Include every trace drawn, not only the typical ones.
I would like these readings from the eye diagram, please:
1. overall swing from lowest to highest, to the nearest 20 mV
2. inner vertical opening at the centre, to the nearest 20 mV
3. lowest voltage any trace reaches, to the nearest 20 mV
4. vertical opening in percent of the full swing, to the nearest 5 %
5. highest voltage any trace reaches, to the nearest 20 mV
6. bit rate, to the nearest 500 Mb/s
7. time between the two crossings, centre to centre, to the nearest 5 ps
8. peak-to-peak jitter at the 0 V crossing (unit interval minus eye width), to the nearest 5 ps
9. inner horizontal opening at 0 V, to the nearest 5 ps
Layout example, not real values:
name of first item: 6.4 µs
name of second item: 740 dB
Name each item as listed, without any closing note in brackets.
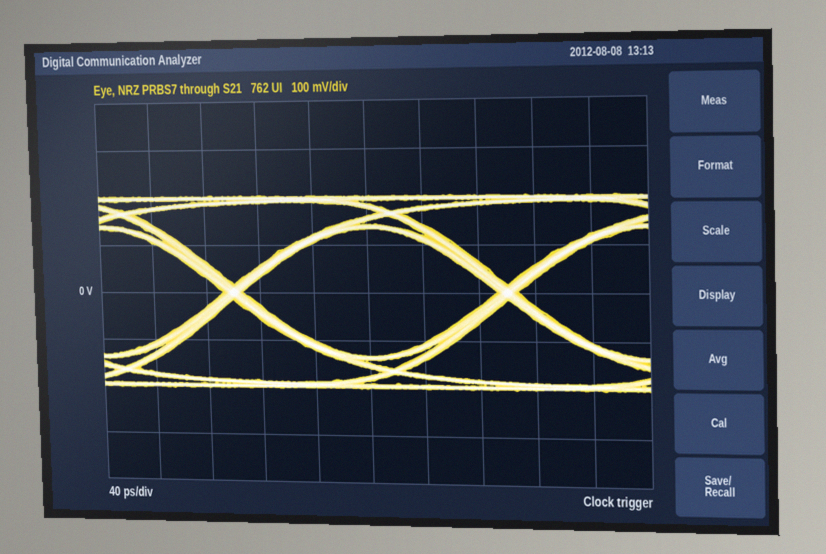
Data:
overall swing from lowest to highest, to the nearest 20 mV: 400 mV
inner vertical opening at the centre, to the nearest 20 mV: 260 mV
lowest voltage any trace reaches, to the nearest 20 mV: -200 mV
vertical opening in percent of the full swing, to the nearest 5 %: 65 %
highest voltage any trace reaches, to the nearest 20 mV: 200 mV
bit rate, to the nearest 500 Mb/s: 5.0 Gb/s
time between the two crossings, centre to centre, to the nearest 5 ps: 200 ps
peak-to-peak jitter at the 0 V crossing (unit interval minus eye width), to the nearest 5 ps: 15 ps
inner horizontal opening at 0 V, to the nearest 5 ps: 185 ps
